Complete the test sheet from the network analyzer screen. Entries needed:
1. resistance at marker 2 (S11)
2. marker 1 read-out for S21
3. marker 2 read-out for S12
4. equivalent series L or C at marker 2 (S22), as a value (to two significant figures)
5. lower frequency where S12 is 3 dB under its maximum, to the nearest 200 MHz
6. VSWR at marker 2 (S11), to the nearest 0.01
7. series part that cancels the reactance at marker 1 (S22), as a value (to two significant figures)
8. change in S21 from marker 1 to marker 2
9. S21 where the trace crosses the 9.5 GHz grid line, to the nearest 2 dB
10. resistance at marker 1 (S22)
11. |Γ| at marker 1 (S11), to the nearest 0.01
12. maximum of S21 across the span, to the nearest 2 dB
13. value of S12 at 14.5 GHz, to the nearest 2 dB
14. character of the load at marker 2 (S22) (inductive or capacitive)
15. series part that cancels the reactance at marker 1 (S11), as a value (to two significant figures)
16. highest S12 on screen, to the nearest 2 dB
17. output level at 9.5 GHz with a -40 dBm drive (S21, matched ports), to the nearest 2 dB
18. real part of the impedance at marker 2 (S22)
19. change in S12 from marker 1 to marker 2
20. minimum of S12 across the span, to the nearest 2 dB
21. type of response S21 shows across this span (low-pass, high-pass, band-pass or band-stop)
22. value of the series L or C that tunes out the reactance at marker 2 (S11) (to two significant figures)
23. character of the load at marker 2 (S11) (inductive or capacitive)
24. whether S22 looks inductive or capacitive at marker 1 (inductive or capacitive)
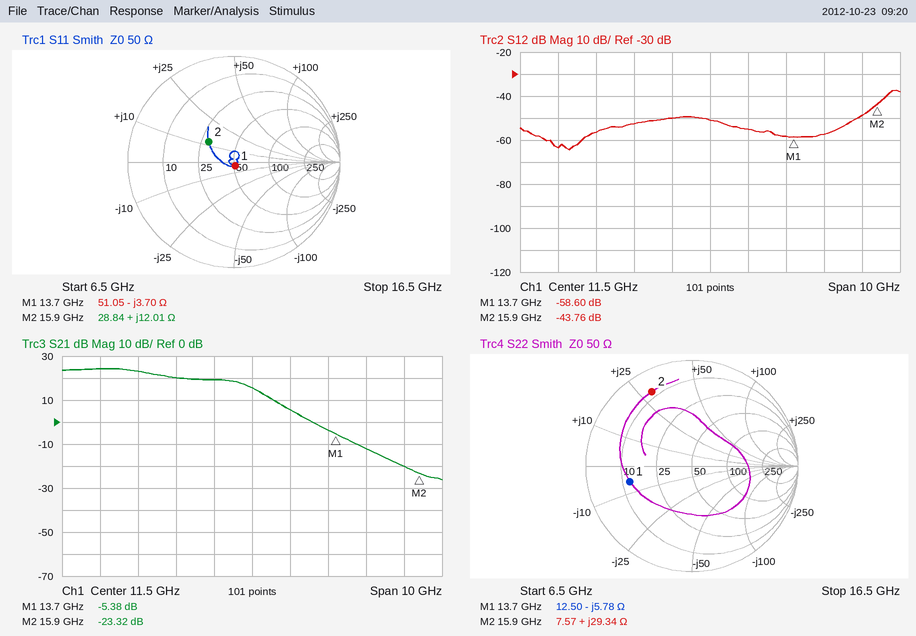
28.84 Ω
-5.38 dB
-43.76 dB
290 pH
16.2 GHz
1.88
67 pH
-17.94 dB
20 dB
12.50 Ω
0.04
24 dB
-58 dB
inductive
43 pH
-38 dB
-20 dBm
7.57 Ω
14.84 dB
-64 dB
low-pass
830 fF
inductive
capacitive
